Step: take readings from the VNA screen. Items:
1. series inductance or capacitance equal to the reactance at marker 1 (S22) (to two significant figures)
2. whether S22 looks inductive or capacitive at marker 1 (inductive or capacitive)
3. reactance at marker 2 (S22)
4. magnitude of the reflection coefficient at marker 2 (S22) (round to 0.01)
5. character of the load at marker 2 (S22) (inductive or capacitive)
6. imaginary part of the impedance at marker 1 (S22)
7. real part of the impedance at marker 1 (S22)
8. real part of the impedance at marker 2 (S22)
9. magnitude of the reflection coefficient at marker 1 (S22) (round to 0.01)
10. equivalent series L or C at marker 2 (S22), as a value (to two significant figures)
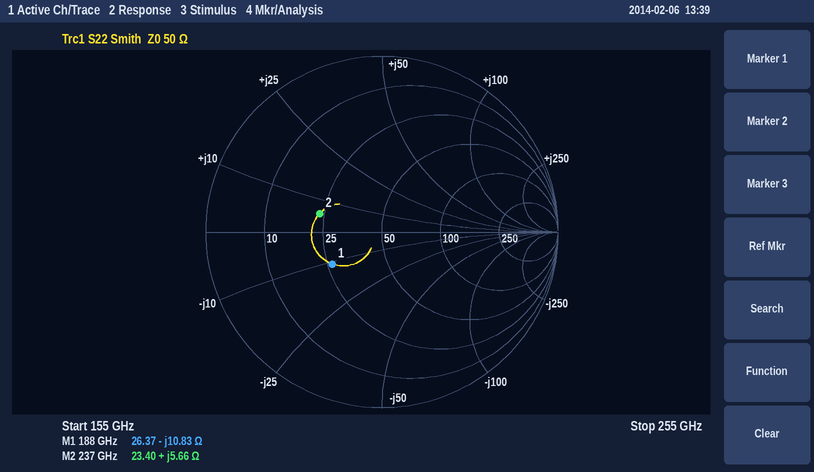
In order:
78 fF
capacitive
+5.66 Ω
0.37
inductive
-10.83 Ω
26.37 Ω
23.40 Ω
0.34
3.8 pH
